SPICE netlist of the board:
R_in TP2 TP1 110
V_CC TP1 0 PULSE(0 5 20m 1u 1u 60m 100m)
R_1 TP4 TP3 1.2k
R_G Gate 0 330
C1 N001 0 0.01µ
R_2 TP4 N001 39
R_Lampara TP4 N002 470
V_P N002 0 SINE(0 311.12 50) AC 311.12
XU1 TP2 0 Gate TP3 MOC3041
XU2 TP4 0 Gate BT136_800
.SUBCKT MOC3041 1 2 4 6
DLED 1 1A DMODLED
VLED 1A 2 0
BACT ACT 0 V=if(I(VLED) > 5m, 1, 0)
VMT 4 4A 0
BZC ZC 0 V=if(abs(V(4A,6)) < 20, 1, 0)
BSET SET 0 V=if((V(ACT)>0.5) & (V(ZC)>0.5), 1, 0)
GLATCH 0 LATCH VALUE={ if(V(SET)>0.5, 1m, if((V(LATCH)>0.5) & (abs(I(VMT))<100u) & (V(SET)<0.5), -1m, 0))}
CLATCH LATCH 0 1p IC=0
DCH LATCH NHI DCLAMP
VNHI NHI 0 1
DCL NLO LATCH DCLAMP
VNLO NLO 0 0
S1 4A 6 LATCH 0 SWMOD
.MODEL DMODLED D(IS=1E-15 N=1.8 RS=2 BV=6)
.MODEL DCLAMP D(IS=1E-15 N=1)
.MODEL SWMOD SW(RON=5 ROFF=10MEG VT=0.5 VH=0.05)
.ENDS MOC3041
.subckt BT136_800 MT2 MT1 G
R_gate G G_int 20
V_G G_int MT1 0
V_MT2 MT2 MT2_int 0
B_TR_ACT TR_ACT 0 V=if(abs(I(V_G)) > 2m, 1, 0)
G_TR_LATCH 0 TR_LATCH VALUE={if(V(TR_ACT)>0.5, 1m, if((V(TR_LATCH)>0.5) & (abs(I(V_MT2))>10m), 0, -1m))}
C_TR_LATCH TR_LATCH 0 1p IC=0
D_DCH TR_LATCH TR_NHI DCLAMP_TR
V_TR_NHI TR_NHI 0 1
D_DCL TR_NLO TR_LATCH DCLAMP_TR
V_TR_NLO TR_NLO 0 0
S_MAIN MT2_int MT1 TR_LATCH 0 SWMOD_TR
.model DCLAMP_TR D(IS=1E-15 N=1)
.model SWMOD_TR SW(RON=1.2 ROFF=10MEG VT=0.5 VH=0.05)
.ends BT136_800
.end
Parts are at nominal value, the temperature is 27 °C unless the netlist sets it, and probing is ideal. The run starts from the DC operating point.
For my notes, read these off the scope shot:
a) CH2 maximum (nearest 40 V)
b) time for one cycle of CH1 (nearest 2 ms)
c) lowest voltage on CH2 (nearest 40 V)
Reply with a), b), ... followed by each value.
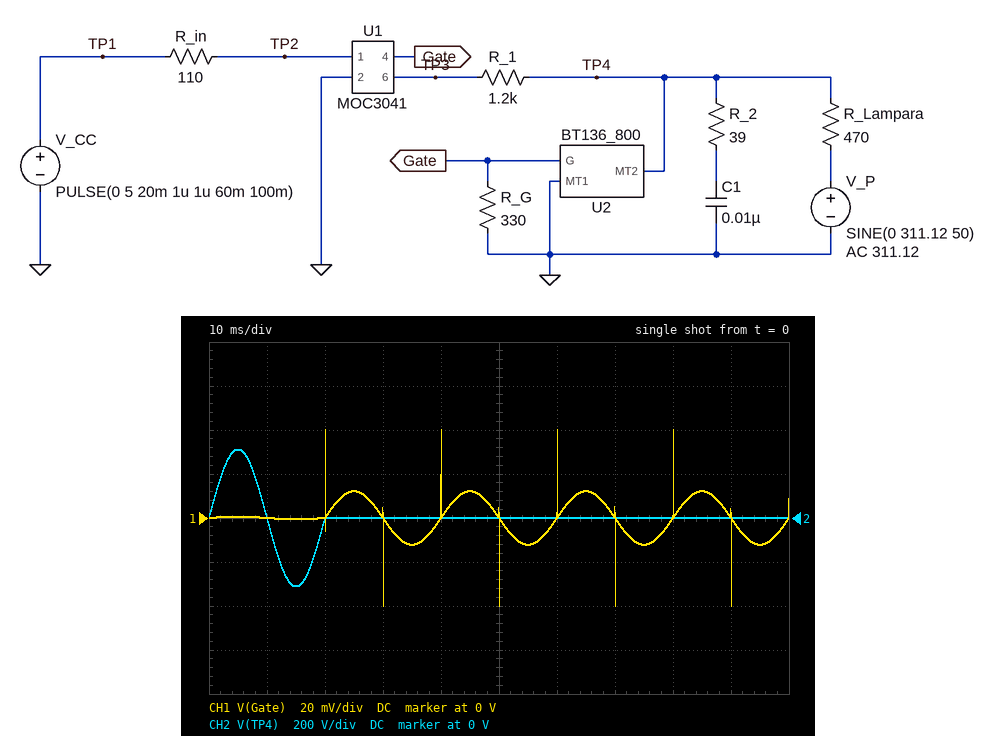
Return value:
a) 320 V
b) 20 ms
c) -320 V
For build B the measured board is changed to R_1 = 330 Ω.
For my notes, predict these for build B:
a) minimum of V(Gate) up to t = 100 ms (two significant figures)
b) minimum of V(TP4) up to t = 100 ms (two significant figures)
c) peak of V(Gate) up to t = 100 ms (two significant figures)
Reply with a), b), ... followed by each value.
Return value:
a) -42 mV
b) -310 V
c) 42 mV
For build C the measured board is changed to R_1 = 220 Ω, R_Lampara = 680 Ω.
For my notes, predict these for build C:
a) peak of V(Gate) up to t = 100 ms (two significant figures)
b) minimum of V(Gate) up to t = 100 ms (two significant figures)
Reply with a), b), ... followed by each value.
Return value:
a) 42 mV
b) -42 mV
